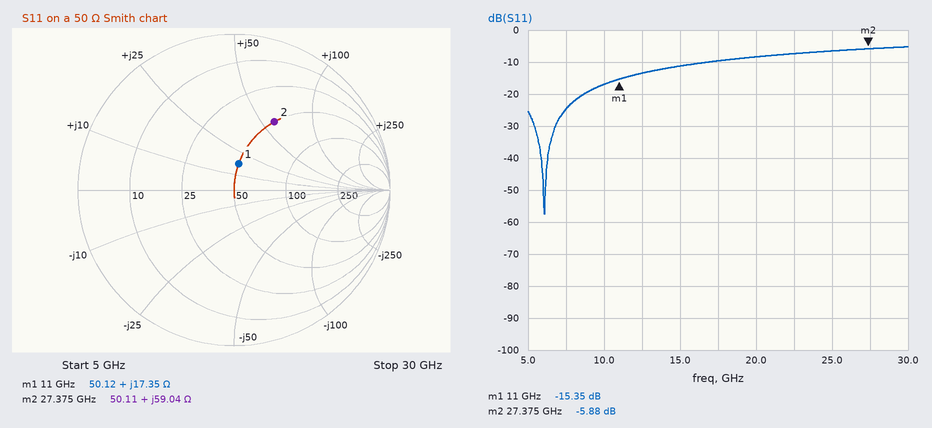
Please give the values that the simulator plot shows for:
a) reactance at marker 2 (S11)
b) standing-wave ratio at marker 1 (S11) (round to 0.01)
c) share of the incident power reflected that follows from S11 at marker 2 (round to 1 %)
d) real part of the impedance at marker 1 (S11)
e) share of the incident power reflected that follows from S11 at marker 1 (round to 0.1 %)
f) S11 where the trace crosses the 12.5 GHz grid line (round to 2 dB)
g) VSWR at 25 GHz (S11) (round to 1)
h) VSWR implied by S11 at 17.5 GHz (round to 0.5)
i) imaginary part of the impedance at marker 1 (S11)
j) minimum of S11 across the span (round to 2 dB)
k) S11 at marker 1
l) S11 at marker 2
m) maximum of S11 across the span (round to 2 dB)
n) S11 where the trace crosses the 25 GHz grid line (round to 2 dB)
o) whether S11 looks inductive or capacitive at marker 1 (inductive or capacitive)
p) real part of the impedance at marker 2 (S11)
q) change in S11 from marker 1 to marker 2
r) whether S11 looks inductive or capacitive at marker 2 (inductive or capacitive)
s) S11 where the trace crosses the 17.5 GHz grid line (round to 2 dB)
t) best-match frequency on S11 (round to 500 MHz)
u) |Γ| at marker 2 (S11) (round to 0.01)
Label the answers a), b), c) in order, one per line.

a) +59.04 Ω
b) 1.41
c) 26 %
d) 50.12 Ω
e) 2.9 %
f) -14 dB
g) 3
h) 2.0
i) +17.35 Ω
j) -58 dB
k) -15.35 dB
l) -5.88 dB
m) -6 dB
n) -6 dB
o) inductive
p) 50.11 Ω
q) 9.47 dB
r) inductive
s) -10 dB
t) 6.0 GHz
u) 0.51
